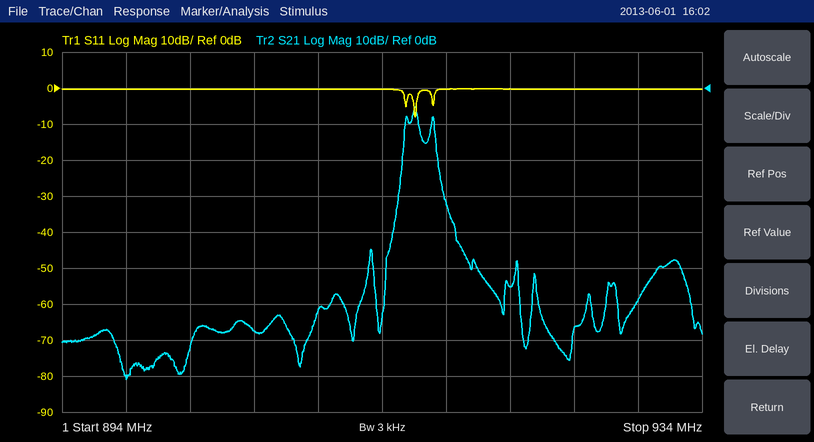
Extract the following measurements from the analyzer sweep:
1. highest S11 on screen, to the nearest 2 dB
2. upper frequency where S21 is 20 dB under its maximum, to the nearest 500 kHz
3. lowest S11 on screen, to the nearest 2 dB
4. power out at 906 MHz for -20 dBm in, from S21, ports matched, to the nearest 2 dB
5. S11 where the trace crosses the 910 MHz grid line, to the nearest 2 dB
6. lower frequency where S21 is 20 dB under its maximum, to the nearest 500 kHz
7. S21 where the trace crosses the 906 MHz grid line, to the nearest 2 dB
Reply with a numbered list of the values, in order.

1. 0 dB
2. 917.5 MHz
3. -8 dB
4. -88 dBm
5. 0 dB
6. 915.0 MHz
7. -68 dB
